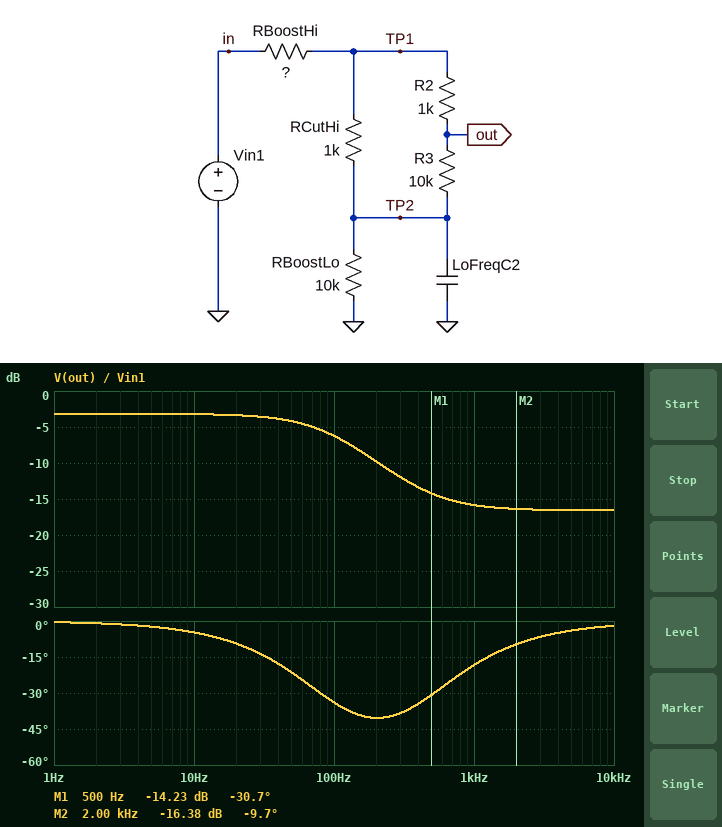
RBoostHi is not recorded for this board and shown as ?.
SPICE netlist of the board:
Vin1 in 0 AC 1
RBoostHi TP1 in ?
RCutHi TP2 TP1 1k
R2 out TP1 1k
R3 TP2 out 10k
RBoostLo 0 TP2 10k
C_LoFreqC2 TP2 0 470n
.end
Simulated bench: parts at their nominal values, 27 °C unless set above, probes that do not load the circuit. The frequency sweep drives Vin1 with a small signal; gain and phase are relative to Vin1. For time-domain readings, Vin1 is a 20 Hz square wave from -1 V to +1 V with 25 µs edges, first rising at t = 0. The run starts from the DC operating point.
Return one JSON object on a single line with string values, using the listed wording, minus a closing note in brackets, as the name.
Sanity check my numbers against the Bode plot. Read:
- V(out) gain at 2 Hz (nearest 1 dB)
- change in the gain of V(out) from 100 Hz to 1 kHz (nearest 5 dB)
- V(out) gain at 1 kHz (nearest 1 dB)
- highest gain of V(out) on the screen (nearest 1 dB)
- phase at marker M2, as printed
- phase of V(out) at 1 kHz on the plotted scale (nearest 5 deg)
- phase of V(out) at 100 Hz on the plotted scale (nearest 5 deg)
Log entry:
{"V(out) gain at 2 Hz": "-3 dB", "change in the gain of V(out) from 100 Hz to 1 kHz": "-10 dB", "V(out) gain at 1 kHz": "-16 dB", "highest gain of V(out) on the screen": "-3 dB", "phase at marker M2, as printed": "-9.7 deg", "phase of V(out) at 1 kHz on the plotted scale": "-20 deg", "phase of V(out) at 100 Hz on the plotted scale": "-35 deg"}
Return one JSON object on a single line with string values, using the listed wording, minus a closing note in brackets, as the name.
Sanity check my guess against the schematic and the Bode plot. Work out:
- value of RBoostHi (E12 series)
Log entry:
{"value of RBoostHi": "4.7 kΩ"}
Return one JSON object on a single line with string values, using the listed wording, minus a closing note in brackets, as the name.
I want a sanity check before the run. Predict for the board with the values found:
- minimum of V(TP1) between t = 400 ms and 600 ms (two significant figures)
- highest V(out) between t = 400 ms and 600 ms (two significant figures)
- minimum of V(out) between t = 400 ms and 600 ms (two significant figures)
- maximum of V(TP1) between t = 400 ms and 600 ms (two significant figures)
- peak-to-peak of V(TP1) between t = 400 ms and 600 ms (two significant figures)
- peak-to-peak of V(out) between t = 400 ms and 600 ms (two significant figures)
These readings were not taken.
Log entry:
{"minimum of V(TP1) between t = 400 ms and 600 ms": "-700 mV", "highest V(out) between t = 400 ms and 600 ms": "690 mV", "minimum of V(out) between t = 400 ms and 600 ms": "-690 mV", "maximum of V(TP1) between t = 400 ms and 600 ms": "700 mV", "peak-to-peak of V(TP1) between t = 400 ms and 600 ms": "1.4 V", "peak-to-peak of V(out) between t = 400 ms and 600 ms": "1.4 V"}
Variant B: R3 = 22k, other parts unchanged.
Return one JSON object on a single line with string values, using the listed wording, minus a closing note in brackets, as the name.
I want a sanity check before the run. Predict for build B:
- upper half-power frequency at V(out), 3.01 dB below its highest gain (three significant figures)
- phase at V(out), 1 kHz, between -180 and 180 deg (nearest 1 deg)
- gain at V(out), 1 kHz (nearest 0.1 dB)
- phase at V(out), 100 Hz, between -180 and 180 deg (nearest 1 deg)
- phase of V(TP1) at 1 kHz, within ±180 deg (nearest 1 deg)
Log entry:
{"upper half-power frequency at V(out), 3.01 dB below its highest gain": "99.2 Hz", "phase at V(out), 1 kHz, between -180 and 180 deg": "-17 deg", "gain at V(out), 1 kHz": "-15.2 dB", "phase at V(out), 100 Hz, between -180 and 180 deg": "-33 deg", "phase of V(TP1) at 1 kHz, within ±180 deg": "-16 deg"}
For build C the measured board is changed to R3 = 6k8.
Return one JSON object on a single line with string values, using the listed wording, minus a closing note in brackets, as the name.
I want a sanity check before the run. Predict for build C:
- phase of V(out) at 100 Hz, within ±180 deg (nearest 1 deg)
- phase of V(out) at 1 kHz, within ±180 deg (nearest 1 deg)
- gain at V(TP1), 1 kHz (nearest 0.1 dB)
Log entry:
{"phase of V(out) at 100 Hz, within ±180 deg": "-35 deg", "phase of V(out) at 1 kHz, within ±180 deg": "-20 deg", "gain at V(TP1), 1 kHz": "-15.3 dB"}
